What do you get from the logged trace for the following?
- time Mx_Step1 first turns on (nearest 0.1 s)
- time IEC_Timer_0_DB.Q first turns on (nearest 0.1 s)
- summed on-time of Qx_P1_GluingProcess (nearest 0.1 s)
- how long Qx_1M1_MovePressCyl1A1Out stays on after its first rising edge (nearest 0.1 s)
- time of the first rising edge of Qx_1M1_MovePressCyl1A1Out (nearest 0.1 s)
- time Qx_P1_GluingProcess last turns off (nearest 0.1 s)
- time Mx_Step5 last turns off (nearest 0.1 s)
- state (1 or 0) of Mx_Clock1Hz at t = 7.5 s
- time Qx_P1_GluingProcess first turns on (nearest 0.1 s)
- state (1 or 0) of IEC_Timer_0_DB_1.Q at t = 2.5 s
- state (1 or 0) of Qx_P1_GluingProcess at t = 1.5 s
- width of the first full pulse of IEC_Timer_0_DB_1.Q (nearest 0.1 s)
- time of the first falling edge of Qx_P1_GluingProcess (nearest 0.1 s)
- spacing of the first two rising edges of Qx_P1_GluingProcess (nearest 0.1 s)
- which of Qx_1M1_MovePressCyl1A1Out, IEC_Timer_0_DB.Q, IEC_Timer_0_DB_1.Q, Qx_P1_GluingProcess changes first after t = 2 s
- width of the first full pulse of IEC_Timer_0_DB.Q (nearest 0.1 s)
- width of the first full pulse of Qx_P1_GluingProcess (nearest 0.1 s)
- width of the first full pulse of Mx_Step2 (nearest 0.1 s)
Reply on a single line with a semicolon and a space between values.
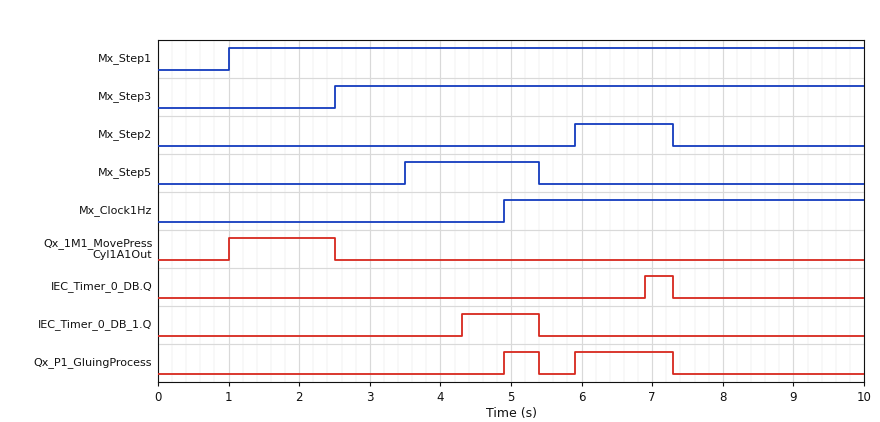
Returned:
1.0 s; 6.9 s; 1.9 s; 1.5 s; 1.0 s; 7.3 s; 5.4 s; 1; 4.9 s; 0; 0; 1.1 s; 5.4 s; 1.0 s; Qx_1M1_MovePressCyl1A1Out; 0.4 s; 0.5 s; 1.4 s
